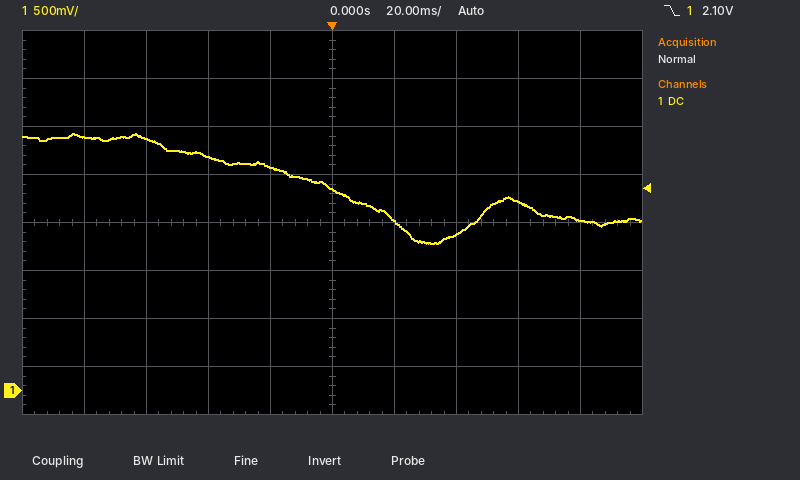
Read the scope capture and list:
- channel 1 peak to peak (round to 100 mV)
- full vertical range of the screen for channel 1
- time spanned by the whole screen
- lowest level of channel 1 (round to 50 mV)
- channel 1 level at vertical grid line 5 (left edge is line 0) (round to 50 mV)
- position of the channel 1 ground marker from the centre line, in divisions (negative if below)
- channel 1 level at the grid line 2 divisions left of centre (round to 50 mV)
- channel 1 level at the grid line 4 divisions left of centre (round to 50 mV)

1.10 V
4 V
200 ms
1.55 V
2.10 V
-3.5 div
2.45 V
2.65 V
